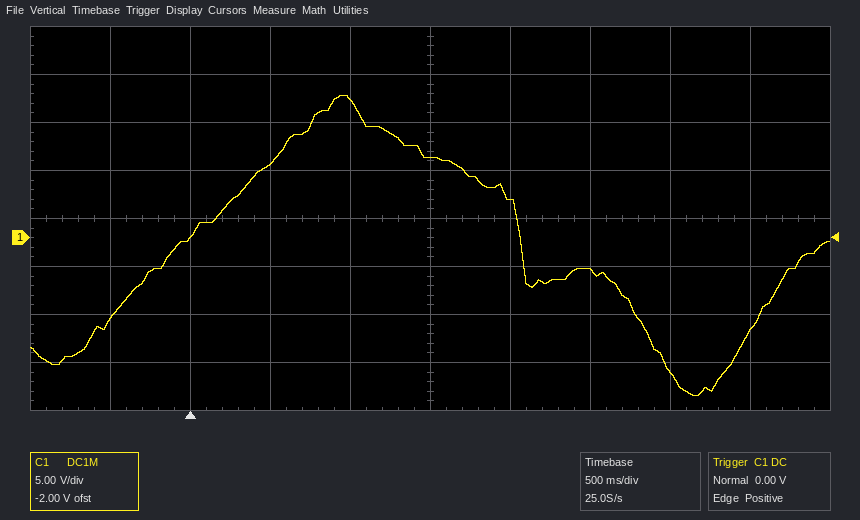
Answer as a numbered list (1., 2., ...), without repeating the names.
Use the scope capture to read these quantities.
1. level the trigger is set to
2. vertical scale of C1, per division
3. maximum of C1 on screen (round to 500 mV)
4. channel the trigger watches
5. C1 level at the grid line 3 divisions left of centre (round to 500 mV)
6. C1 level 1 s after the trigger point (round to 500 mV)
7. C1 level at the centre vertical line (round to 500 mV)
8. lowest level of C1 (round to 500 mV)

1. 0.00 V
2. 5 V
3. 15.0 V
4. C1
5. 0.0 V
6. 14.5 V
7. 8.5 V
8. -16.5 V
